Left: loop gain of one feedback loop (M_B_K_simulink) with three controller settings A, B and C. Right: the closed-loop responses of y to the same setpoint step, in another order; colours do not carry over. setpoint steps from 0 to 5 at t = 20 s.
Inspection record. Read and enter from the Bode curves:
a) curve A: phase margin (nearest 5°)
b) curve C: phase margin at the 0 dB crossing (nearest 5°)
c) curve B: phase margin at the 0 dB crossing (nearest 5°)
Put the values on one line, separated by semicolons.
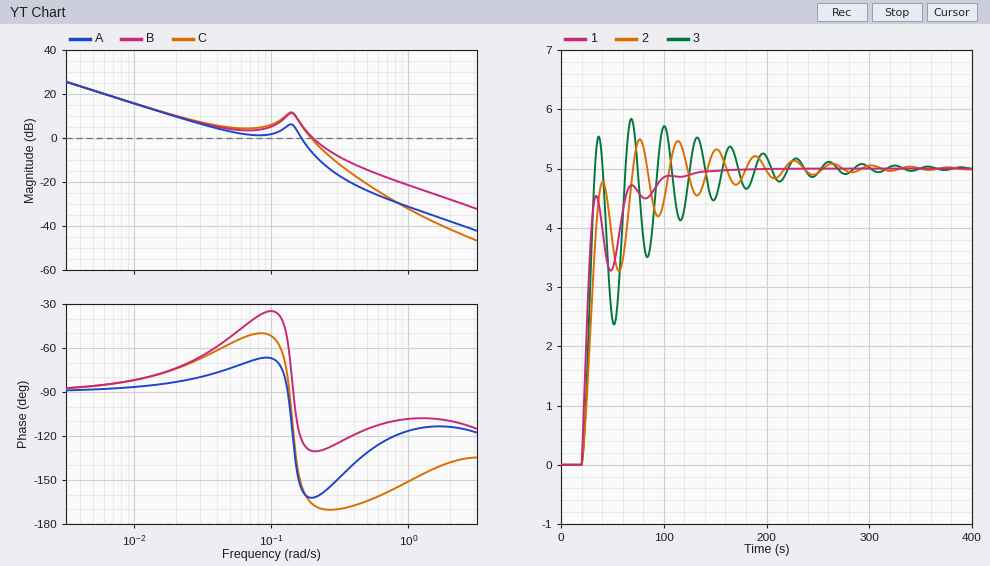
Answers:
25°; 15°; 50°
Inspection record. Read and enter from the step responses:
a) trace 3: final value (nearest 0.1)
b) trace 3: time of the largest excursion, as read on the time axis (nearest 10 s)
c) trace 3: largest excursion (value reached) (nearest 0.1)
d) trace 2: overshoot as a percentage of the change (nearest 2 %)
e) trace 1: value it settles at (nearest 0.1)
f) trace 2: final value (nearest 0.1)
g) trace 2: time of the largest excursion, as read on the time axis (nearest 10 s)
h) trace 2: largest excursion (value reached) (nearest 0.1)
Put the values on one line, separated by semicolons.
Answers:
5.0; 70 s; 5.8; 10 %; 5.0; 5.0; 80 s; 5.5
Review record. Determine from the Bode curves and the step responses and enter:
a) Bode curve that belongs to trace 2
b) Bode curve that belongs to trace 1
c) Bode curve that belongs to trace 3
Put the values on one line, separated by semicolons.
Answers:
A; B; C
